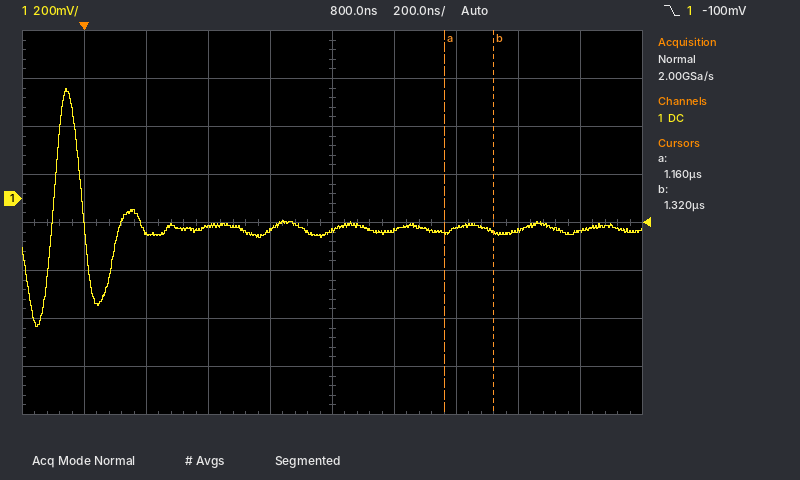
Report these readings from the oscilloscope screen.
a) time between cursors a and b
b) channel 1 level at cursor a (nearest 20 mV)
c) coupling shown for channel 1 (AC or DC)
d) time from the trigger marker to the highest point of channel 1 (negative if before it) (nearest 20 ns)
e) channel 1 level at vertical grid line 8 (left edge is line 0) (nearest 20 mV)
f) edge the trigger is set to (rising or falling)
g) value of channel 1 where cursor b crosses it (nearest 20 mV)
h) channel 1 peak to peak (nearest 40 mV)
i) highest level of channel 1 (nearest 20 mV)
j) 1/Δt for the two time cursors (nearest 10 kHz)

160 ns
-140 mV
DC
-60 ns
-140 mV
falling
-140 mV
1.00 V
460 mV
6.25 MHz
